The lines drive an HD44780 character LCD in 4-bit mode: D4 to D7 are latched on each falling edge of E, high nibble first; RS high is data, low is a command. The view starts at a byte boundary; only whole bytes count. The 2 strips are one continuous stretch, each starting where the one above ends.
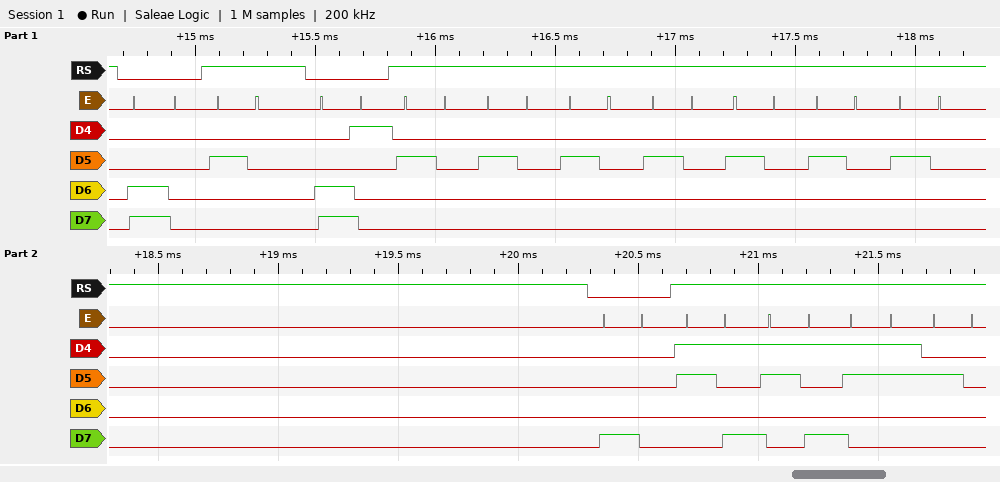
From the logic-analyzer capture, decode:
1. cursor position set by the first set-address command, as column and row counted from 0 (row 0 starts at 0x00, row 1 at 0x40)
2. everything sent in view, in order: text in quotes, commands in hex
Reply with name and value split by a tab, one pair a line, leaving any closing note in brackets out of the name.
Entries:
cursor position set by the first set-address command, as column and row counted from 0	column 0, row 1
everything sent in view, in order: text in quotes, commands in hex	0xC0 " " 0xC1 "       " 0x80 "993 "
